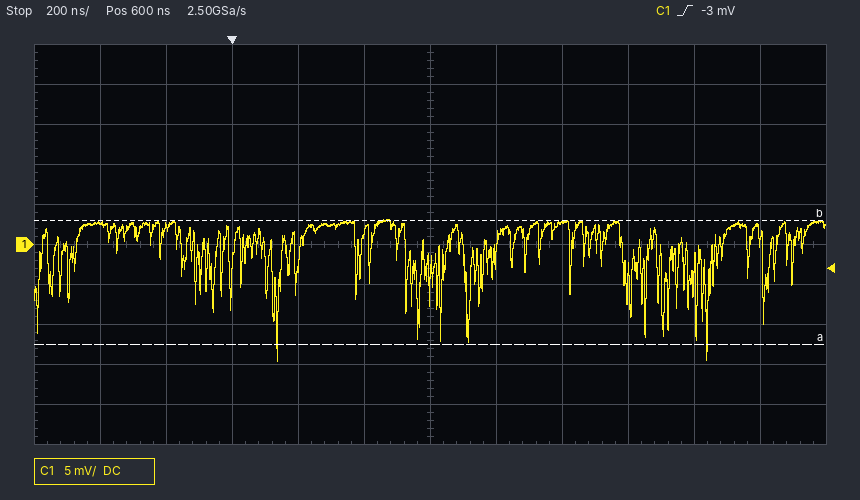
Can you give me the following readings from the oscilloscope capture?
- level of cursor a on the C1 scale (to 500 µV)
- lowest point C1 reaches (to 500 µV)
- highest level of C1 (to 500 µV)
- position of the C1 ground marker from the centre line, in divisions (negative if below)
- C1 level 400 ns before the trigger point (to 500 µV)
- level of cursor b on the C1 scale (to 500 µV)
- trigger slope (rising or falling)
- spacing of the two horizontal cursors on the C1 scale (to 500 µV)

-12.5 mV
-14.5 mV
3.0 mV
0.0 div
2.5 mV
3.0 mV
rising
15.5 mV
